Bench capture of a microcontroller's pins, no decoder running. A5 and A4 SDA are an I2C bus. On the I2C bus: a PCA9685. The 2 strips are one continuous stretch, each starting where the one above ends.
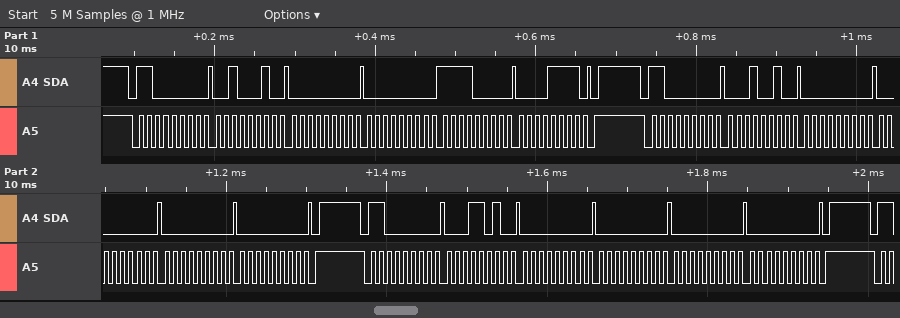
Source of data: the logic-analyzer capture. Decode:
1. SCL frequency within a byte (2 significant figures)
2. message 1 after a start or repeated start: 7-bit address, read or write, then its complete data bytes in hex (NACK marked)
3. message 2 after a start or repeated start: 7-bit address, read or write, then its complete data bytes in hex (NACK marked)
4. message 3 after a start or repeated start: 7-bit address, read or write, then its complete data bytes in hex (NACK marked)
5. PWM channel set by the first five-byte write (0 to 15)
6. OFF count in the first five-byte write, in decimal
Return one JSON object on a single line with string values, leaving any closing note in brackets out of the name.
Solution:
{"SCL frequency within a byte": "100 kHz", "message 1 after a start or repeated start: 7-bit address, read or write, then its complete data bytes in hex": "0x60 write: 22 00 00 F0 0F", "message 2 after a start or repeated start: 7-bit address, read or write, then its complete data bytes in hex": "0x60 write: 12 00 00 00 00", "message 3 after a start or repeated start: 7-bit address, read or write, then its complete data bytes in hex": "0x60 write: 1A 00 00 00 00", "PWM channel set by the first five-byte write": "7", "OFF count in the first five-byte write, in decimal": "4080"}
